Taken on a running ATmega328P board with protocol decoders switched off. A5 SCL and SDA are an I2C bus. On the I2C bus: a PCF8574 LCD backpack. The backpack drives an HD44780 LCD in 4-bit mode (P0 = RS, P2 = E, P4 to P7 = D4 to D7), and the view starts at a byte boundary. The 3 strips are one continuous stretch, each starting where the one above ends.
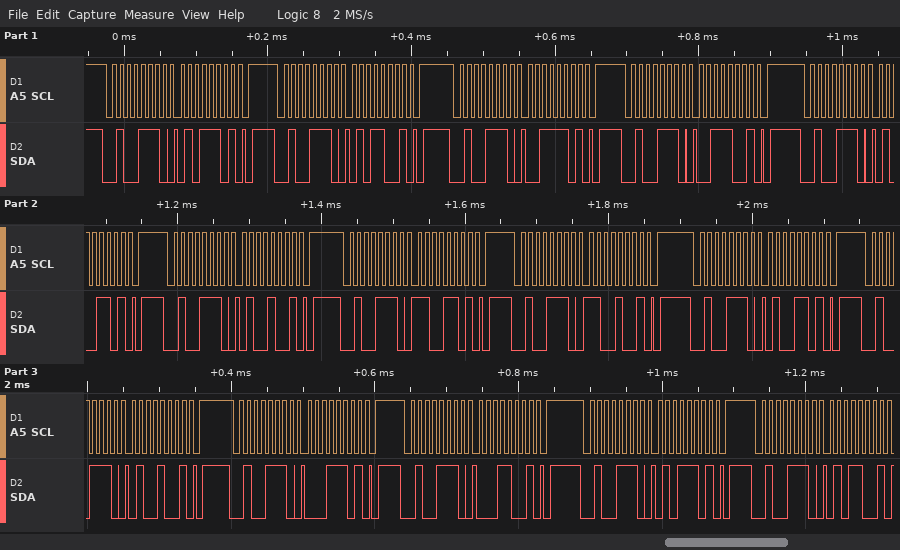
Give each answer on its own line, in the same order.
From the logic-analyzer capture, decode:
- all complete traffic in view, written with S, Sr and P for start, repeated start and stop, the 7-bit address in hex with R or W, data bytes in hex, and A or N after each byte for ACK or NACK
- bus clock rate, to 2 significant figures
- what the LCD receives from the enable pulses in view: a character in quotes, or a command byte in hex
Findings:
S 27W A 5D A P S 27W A 59 A P S 27W A 3D A P S 27W A 39 A P S 27W A 4D A P S 27W A 49 A P S 27W A CD A P S 27W A C9 A P S 27W A 4D A P S 27W A 49 A P S 27W A 1D A P S 27W A 19 A P S 27W A 5D A P S 27W A 59 A
100 kHz
'S' 'L' 'A'
